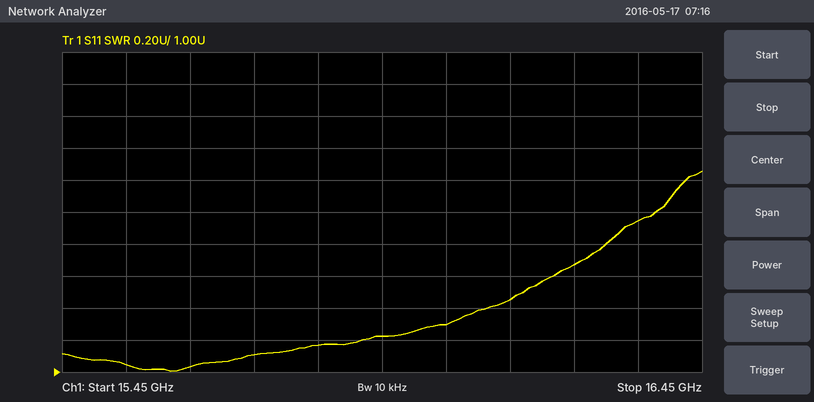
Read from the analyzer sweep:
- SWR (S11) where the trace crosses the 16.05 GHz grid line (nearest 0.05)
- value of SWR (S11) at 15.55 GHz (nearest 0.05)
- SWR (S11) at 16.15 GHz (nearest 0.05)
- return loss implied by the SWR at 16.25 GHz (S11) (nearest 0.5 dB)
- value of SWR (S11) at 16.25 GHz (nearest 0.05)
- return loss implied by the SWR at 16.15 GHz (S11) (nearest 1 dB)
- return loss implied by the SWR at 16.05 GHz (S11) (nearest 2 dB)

1.30
1.05
1.45
12.0 dB
1.65
15 dB
18 dB
